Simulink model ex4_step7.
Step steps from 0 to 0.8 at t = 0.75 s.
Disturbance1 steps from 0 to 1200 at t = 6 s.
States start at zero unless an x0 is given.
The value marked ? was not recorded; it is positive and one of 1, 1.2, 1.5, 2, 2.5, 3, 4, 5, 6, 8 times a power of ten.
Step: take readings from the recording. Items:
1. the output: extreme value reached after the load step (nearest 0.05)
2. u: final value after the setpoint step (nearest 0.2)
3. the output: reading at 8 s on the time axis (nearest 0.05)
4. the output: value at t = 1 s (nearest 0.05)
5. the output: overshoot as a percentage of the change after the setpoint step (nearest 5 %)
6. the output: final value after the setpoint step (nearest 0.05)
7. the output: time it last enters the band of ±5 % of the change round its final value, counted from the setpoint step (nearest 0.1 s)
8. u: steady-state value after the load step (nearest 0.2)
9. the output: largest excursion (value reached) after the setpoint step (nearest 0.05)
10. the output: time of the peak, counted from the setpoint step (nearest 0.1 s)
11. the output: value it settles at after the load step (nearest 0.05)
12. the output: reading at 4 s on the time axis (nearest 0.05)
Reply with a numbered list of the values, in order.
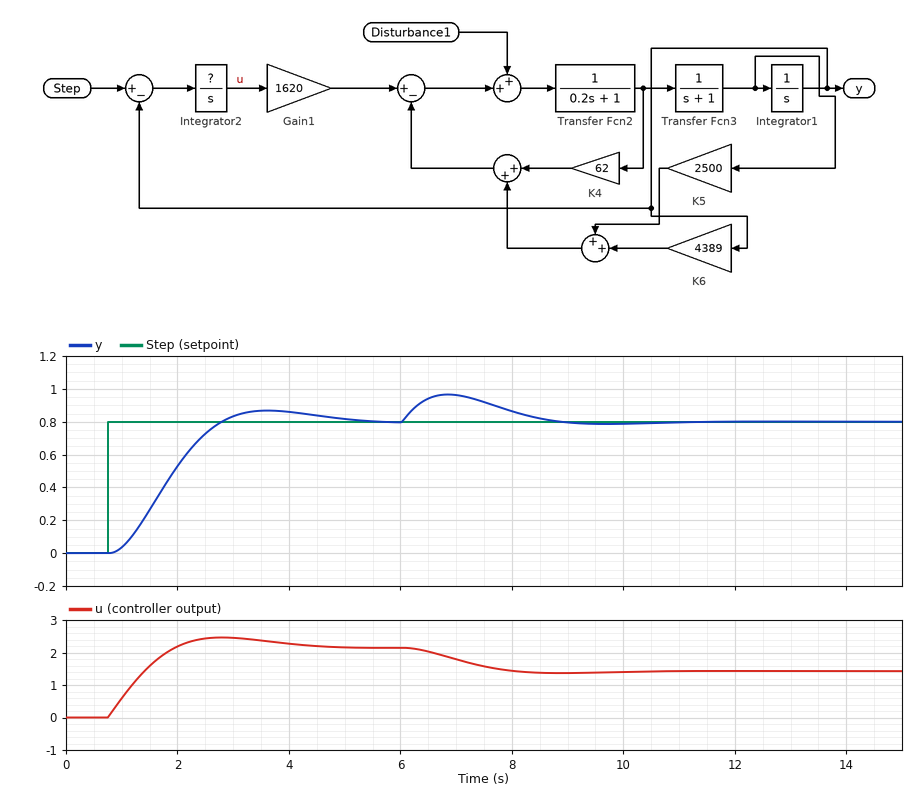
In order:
1. 0.95
2. 2.2
3. 0.85
4. 0.05
5. 10 %
6. 0.80
7. 3.7 s
8. 1.4
9. 0.85
10. 2.9 s
11. 0.80
12. 0.85
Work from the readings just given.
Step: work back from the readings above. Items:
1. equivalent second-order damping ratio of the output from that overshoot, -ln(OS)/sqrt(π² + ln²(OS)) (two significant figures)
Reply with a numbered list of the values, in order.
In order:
1. 0.59
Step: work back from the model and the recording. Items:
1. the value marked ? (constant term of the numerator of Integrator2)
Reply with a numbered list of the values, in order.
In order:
1. 3
